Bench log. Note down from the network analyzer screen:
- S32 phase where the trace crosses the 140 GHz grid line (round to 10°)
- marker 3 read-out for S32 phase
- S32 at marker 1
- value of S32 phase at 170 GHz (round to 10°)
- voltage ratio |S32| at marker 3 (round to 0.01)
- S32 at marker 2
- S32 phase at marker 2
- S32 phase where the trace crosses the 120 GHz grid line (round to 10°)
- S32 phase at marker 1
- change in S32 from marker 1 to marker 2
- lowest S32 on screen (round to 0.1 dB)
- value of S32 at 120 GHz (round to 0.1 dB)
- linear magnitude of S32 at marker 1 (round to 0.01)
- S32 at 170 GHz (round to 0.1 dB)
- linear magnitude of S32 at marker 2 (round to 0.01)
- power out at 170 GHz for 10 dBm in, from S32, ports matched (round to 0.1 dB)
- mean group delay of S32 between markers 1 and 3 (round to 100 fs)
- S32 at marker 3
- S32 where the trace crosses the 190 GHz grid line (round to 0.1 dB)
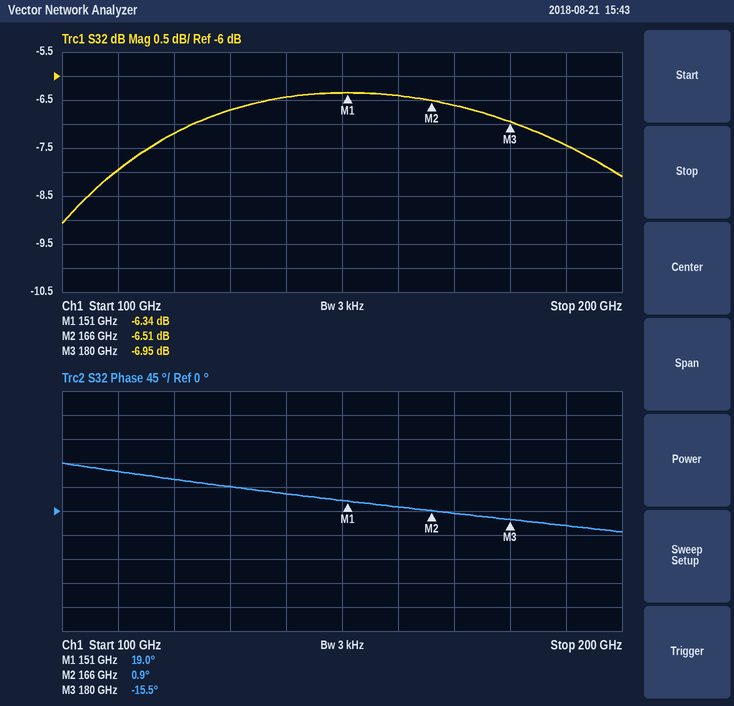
30°
-15.5°
-6.34 dB
0°
0.45
-6.51 dB
0.9°
60°
19.0°
-0.17 dB
-9.1 dB
-7.2 dB
0.48
-6.6 dB
0.47
3.4 dBm
3.3 ps
-6.95 dB
-7.4 dB
